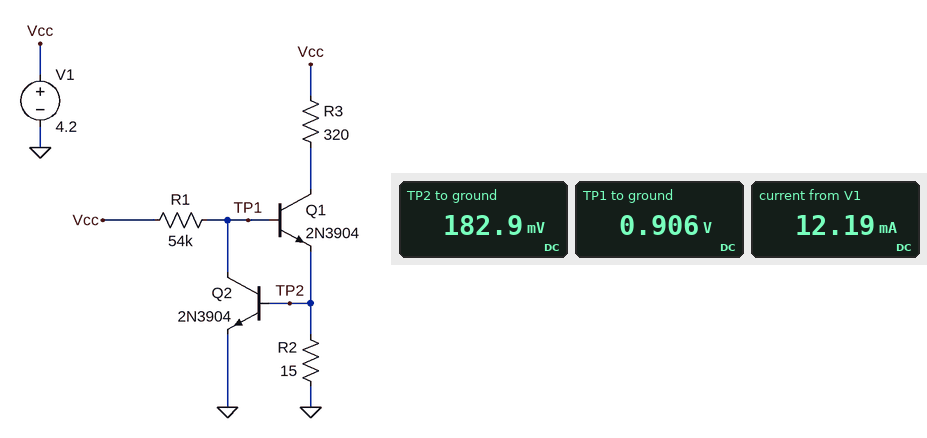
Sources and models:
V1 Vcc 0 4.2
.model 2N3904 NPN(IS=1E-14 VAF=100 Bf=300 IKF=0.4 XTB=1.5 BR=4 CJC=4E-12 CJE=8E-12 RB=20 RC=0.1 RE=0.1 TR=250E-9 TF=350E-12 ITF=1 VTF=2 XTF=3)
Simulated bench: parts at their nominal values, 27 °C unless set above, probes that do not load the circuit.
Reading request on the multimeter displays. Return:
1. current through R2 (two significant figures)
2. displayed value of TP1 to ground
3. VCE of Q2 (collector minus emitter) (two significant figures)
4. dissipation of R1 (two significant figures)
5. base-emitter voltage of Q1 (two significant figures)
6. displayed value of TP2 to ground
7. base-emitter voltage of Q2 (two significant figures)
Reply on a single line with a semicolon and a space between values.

12 mA; 0.906 V; 910 mV; 200 µW; 720 mV; 182.9 mV; 180 mV
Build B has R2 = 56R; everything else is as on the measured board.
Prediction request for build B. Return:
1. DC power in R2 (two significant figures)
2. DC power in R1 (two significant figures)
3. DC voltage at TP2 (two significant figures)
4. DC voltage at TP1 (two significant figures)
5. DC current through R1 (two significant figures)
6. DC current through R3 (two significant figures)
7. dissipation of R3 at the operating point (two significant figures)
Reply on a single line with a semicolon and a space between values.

5.5 mW; 160 µW; 550 mV; 1.3 V; 54 µA; 9.9 mA; 31 mW
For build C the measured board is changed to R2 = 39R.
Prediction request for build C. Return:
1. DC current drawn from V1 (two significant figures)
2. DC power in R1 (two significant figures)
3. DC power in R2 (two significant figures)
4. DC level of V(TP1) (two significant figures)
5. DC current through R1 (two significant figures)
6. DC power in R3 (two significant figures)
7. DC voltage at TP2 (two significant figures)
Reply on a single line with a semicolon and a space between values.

11 mA; 170 µW; 5.0 mW; 1.2 V; 56 µA; 41 mW; 440 mV
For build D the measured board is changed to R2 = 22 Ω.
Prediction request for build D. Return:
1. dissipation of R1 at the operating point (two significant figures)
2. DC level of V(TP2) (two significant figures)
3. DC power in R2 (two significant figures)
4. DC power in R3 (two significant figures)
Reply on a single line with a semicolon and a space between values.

190 µW; 260 mV; 3.1 mW; 45 mW
